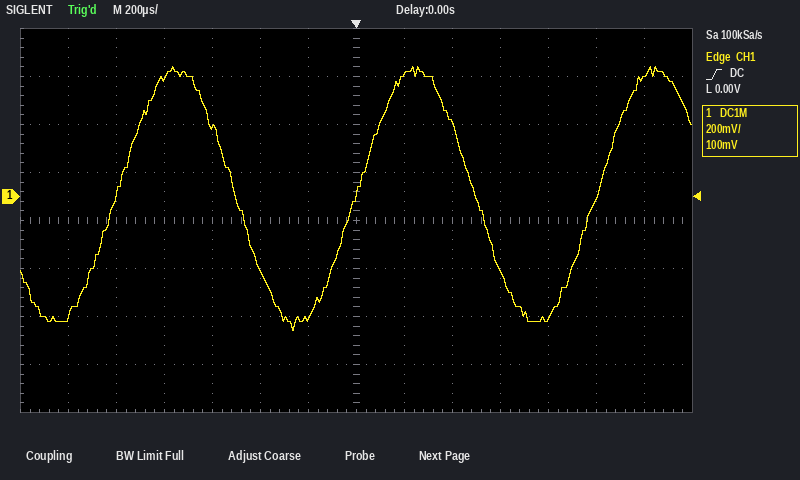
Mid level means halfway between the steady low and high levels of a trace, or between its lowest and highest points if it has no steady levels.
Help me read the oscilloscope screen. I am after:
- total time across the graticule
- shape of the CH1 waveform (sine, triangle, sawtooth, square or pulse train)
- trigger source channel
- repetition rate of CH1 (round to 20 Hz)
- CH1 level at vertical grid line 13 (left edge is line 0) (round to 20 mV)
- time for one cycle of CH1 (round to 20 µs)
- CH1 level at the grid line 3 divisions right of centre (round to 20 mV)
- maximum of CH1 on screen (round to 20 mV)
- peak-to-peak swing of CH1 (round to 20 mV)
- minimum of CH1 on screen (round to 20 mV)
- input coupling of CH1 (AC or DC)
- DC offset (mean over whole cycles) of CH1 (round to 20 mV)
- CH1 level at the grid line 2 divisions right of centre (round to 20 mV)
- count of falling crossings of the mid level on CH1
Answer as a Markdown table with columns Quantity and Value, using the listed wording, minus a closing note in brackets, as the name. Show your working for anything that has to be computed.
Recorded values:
| Quantity | Value |
|---|---|
| total time across the graticule | 2.8 ms |
| shape of the CH1 waveform | sine |
| trigger source channel | CH1 |
| repetition rate of CH1 | 1 / 1.00 ms ≈ 1.00 kHz |
| CH1 level at vertical grid line 13 (left edge is line 0) | 500 mV |
| time for one cycle of CH1 | 1.00 ms |
| CH1 level at the grid line 3 divisions right of centre | -300 mV |
| maximum of CH1 on screen | 540 mV |
| peak-to-peak swing of CH1 | 540 mV − (-560 mV) = 1.10 V |
| minimum of CH1 on screen | -560 mV |
| input coupling of CH1 | DC |
| DC offset (mean over whole cycles) of CH1 | (540 mV + (-560 mV)) / 2 ≈ 0 mV |
| CH1 level at the grid line 2 divisions right of centre | 300 mV |
| count of falling crossings of the mid level on CH1 | 2 |
